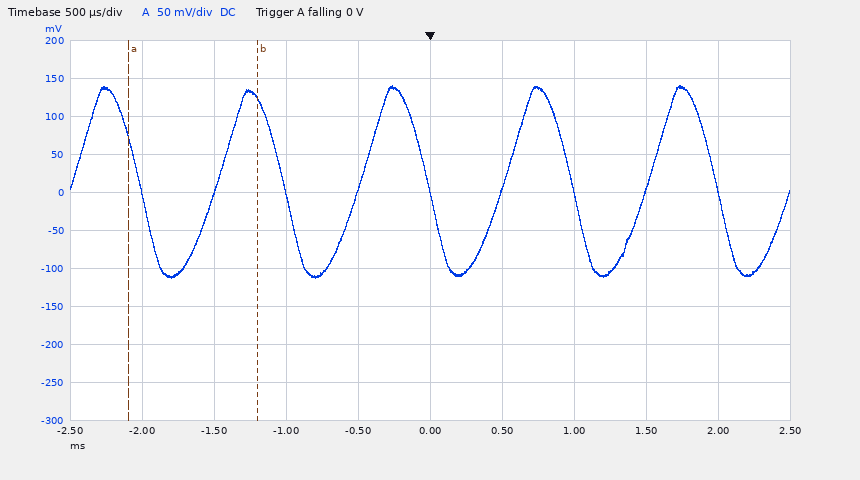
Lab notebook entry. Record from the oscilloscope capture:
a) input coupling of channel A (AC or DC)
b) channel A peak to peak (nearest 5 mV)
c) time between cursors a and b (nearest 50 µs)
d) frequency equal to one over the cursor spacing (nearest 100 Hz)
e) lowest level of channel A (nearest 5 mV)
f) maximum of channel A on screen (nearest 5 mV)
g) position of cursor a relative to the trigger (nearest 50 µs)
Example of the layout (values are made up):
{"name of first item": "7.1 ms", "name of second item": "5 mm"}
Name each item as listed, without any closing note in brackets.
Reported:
{"input coupling of channel A": "DC", "channel A peak to peak": "255 mV", "time between cursors a and b": "900 µs", "frequency equal to one over the cursor spacing": "1.1 kHz", "lowest level of channel A": "-115 mV", "maximum of channel A on screen": "140 mV", "position of cursor a relative to the trigger": "-2.10 ms"}
